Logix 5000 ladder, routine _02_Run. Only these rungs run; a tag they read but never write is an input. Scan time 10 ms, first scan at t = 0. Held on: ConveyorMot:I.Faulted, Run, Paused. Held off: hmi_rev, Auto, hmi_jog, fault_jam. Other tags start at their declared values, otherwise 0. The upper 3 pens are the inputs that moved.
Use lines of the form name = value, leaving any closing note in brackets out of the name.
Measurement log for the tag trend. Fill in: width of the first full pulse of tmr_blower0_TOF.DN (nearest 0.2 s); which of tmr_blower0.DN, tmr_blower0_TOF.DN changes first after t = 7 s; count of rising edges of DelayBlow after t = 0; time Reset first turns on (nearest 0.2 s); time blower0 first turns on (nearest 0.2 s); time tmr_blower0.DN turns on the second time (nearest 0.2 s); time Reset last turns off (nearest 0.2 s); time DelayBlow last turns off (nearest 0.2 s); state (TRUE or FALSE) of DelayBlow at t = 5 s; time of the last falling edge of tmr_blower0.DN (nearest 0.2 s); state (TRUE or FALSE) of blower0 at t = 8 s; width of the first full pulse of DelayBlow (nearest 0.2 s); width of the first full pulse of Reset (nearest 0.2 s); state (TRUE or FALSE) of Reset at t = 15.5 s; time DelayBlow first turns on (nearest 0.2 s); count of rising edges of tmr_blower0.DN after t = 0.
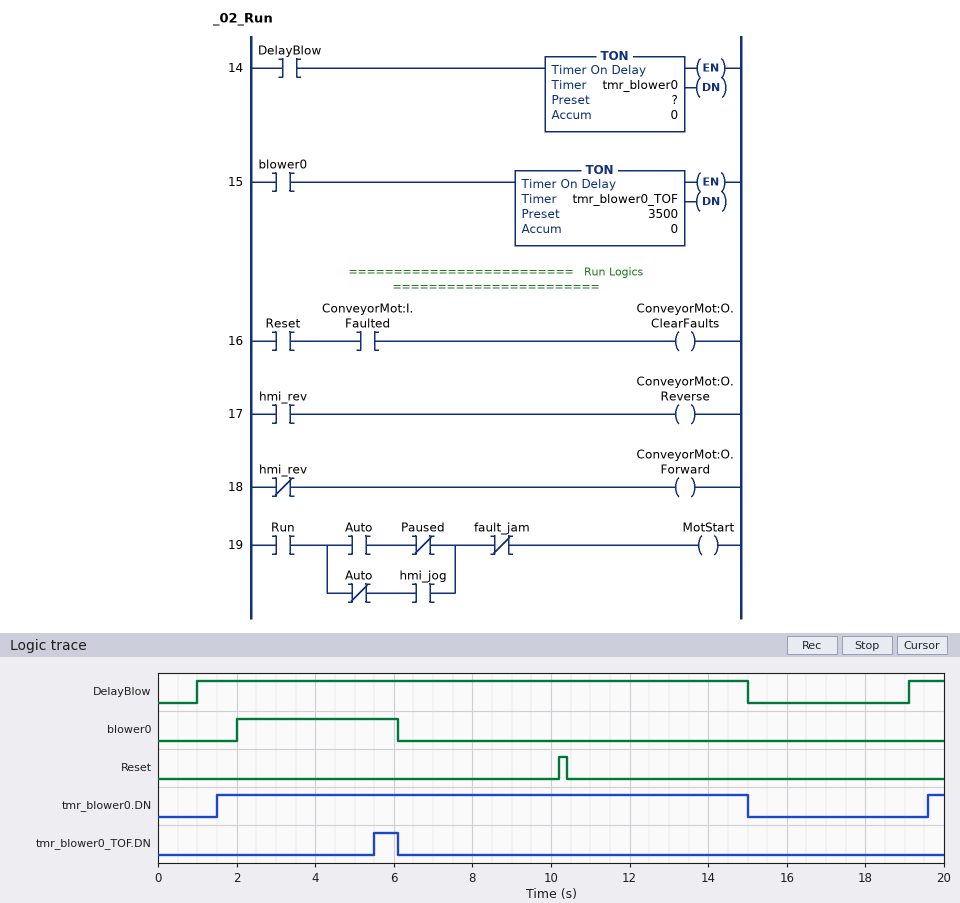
width of the first full pulse of tmr_blower0_TOF.DN = 0.6 s
which of tmr_blower0.DN, tmr_blower0_TOF.DN changes first after t = 7 s = tmr_blower0.DN
count of rising edges of DelayBlow after t = 0 = 2
time Reset first turns on = 10.2 s
time blower0 first turns on = 2.0 s
time tmr_blower0.DN turns on the second time = 19.6 s
time Reset last turns off = 10.4 s
time DelayBlow last turns off = 15.0 s
state (TRUE or FALSE) of DelayBlow at t = 5 s = TRUE
time of the last falling edge of tmr_blower0.DN = 15.0 s
state (TRUE or FALSE) of blower0 at t = 8 s = FALSE
width of the first full pulse of DelayBlow = 14.0 s
width of the first full pulse of Reset = 0.2 s
state (TRUE or FALSE) of Reset at t = 15.5 s = FALSE
time DelayBlow first turns on = 1.0 s
count of rising edges of tmr_blower0.DN after t = 0 = 2
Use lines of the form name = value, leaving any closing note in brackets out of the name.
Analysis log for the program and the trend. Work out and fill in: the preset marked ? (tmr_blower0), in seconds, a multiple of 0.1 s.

the preset marked ? (tmr_blower0), in seconds, a multiple of 0.1 s = 0.5 s
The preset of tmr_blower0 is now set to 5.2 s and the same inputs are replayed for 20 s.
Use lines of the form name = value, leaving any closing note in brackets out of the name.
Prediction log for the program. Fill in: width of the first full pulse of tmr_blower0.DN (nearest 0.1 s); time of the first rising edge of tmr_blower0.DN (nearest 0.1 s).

width of the first full pulse of tmr_blower0.DN = 8.8 s
time of the first rising edge of tmr_blower0.DN = 6.2 s
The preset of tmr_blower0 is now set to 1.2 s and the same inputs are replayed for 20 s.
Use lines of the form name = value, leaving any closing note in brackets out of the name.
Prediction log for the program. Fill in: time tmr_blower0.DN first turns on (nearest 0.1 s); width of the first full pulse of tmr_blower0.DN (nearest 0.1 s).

time tmr_blower0.DN first turns on = 2.2 s
width of the first full pulse of tmr_blower0.DN = 12.8 s
